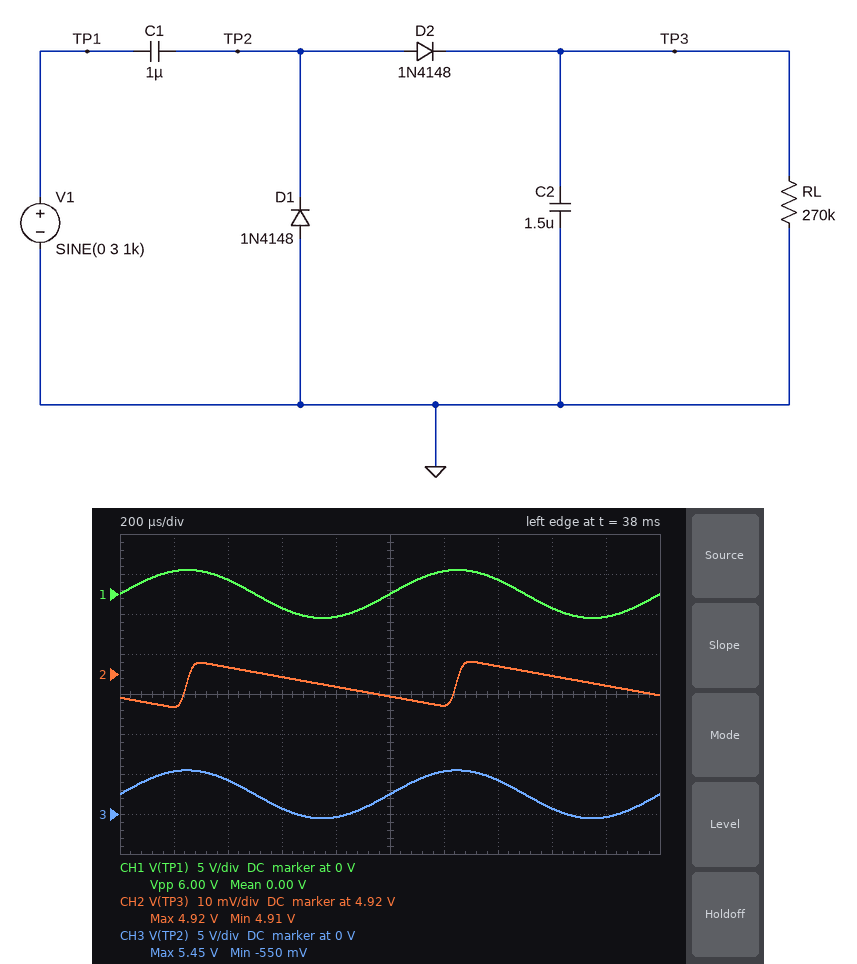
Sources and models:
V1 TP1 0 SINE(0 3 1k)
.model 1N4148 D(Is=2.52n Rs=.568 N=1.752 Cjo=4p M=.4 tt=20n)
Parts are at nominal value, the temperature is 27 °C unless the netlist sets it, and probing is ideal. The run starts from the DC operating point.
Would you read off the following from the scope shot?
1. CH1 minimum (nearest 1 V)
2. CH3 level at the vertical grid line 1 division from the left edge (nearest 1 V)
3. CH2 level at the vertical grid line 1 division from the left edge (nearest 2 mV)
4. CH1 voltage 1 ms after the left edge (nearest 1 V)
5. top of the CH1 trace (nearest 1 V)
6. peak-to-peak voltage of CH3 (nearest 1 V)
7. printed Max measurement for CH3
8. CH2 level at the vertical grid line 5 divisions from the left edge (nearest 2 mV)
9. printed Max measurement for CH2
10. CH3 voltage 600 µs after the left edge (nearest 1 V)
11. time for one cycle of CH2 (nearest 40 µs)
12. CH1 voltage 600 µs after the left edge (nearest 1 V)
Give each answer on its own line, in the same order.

-3 V
5 V
4.912 V
0 V
3 V
6 V
5.45 V
4.914 V
4.92 V
1 V
1.00 ms
-2 V
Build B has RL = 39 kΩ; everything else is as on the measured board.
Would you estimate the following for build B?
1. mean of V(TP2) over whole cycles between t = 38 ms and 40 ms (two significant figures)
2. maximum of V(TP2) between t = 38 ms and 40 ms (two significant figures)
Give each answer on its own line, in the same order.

2.4 V
5.3 V
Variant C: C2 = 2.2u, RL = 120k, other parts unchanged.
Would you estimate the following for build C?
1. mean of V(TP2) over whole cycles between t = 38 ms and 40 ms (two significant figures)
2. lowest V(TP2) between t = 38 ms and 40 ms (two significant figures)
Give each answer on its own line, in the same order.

2.4 V
-580 mV
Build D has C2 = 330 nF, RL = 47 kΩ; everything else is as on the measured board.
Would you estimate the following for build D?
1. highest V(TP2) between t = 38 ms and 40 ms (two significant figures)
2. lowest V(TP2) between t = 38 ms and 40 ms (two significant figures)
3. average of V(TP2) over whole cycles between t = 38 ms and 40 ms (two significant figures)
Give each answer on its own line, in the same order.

5.3 V
-620 mV
2.4 V
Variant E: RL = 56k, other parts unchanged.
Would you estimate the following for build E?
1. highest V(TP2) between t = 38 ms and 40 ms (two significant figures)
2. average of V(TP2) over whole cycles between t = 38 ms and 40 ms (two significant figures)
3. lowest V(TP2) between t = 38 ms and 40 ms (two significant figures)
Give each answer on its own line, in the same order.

5.4 V
2.4 V
-610 mV
